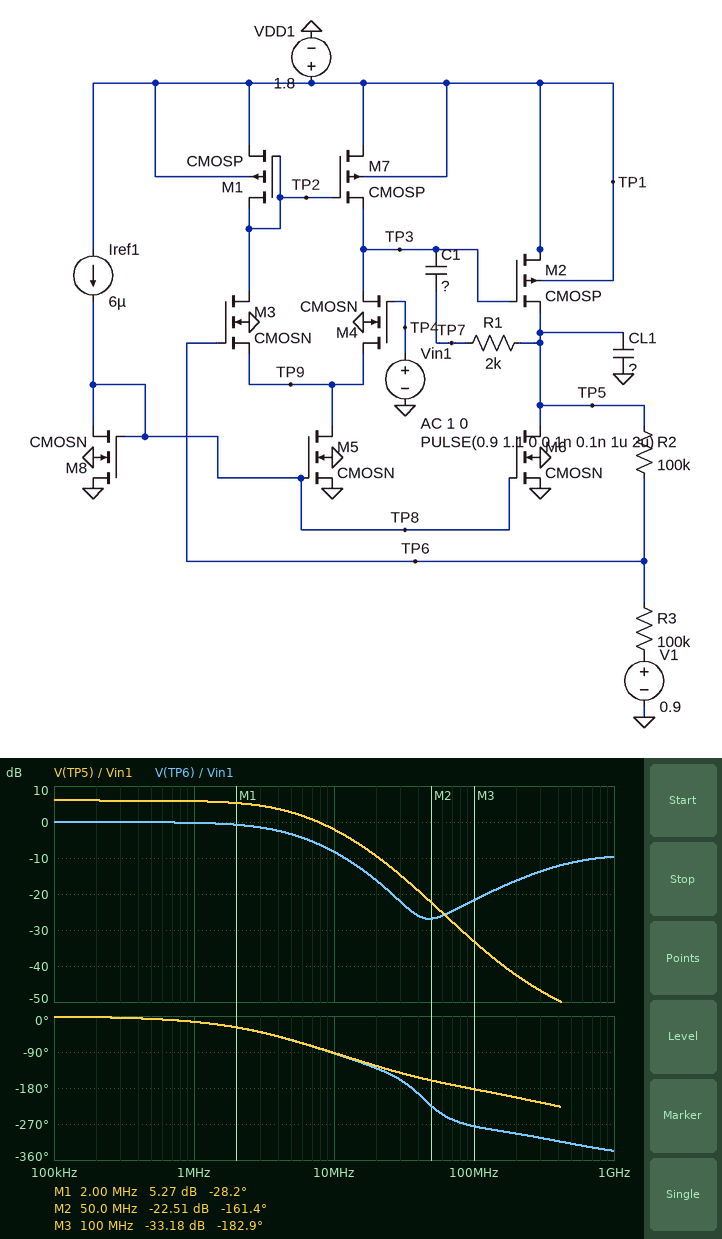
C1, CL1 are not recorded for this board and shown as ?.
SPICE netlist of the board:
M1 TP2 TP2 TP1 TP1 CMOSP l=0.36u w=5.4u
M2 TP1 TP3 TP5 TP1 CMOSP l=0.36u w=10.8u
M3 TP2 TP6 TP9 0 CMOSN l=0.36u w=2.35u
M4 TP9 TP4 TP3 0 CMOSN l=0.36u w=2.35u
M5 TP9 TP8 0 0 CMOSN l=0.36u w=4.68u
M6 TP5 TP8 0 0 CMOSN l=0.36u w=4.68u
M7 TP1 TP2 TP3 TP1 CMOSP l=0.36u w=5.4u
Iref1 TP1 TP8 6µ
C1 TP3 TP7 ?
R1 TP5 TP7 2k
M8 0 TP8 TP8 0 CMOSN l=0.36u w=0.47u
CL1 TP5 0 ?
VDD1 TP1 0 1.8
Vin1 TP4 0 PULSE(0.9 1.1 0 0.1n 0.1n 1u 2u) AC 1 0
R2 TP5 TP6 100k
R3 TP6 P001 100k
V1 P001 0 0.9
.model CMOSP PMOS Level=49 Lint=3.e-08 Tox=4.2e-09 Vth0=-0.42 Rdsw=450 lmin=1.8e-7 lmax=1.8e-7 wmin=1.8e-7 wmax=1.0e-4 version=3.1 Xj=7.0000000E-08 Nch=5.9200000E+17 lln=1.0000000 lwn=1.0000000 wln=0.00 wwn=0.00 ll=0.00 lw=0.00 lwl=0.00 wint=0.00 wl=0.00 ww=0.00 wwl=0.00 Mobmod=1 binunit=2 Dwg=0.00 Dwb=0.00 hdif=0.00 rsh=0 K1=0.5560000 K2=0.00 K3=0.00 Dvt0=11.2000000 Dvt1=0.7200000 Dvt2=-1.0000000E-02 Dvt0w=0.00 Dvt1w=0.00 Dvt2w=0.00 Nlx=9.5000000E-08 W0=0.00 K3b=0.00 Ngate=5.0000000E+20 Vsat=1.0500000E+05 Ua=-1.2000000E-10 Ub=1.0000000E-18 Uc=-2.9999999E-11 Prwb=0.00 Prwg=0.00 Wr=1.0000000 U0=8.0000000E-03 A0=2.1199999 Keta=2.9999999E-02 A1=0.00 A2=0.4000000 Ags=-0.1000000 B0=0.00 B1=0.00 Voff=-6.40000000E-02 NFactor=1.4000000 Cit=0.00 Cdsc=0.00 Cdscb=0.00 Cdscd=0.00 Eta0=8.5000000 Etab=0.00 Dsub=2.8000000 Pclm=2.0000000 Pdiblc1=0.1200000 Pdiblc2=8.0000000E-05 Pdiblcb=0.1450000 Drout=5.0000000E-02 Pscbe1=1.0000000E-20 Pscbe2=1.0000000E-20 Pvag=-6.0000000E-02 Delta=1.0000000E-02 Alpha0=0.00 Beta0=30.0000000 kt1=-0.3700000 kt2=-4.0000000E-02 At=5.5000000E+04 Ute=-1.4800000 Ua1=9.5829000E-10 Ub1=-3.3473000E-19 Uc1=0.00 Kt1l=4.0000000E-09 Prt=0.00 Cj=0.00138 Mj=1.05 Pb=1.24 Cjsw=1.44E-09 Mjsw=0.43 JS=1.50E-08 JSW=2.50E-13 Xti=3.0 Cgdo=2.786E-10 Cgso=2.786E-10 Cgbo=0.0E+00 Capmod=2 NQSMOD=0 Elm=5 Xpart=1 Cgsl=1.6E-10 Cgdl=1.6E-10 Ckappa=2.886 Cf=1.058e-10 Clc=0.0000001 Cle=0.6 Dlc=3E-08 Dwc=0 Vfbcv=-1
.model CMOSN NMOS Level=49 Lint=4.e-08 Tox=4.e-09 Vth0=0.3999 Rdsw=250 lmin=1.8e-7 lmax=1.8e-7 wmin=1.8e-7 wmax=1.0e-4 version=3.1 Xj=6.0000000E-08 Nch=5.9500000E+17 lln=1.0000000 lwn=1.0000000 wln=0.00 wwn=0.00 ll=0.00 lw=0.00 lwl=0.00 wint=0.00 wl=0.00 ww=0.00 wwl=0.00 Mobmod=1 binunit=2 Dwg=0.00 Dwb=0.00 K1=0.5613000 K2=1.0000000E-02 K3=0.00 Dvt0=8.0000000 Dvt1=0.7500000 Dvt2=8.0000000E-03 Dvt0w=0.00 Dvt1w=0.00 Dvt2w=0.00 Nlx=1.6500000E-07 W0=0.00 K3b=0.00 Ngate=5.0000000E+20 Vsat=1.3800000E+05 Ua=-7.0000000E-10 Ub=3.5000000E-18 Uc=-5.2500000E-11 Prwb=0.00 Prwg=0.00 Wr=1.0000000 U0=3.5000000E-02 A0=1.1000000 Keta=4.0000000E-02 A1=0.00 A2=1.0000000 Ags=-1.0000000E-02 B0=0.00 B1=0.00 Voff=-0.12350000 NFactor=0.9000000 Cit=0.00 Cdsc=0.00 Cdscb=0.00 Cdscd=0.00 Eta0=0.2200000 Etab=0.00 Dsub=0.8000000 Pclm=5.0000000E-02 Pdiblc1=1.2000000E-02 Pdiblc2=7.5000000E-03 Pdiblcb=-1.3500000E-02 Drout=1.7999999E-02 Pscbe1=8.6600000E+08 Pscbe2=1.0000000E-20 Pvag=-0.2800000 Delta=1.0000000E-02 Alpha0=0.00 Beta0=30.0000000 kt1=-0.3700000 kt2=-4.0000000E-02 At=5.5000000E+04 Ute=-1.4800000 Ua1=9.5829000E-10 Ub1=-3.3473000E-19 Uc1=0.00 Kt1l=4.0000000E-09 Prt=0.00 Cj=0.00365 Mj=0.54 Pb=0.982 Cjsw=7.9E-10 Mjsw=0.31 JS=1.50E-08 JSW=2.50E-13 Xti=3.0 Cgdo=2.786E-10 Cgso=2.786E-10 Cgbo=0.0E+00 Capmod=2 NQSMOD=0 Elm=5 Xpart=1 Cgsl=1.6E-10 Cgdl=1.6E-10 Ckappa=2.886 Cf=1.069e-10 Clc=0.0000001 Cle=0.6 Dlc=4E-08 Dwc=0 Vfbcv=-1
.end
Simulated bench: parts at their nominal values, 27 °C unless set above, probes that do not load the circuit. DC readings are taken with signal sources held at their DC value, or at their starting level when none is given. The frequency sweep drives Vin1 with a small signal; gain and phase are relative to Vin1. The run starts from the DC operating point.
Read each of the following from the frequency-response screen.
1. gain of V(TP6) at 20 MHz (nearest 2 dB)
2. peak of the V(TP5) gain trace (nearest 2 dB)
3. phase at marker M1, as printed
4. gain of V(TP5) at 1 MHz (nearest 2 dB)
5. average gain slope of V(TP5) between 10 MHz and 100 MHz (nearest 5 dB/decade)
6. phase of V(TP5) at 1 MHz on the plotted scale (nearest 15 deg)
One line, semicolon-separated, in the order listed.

-16 dB; 6 dB; -28.2 deg; 6 dB; -30 dB/decade; -15 deg
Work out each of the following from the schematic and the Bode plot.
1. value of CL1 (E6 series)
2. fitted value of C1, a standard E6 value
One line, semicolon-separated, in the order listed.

3.3 pF; 4.7 pF
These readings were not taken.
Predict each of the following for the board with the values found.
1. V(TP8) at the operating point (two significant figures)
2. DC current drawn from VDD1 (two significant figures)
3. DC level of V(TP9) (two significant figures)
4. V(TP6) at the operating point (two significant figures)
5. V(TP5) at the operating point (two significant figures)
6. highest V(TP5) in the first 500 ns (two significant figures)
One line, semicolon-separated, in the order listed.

680 mV; 120 µA; 180 mV; 900 mV; 900 mV; 1.3 V
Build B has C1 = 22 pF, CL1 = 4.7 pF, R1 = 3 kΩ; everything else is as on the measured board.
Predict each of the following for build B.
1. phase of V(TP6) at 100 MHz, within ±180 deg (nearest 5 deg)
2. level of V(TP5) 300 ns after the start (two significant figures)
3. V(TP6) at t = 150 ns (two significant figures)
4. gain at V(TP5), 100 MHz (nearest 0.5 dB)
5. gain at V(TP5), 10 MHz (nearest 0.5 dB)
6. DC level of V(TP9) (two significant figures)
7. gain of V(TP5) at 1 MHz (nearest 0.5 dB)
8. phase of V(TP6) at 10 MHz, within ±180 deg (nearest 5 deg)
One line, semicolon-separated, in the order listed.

80 deg; 1.2 V; 1.0 V; -28.5 dB; -12.5 dB; 180 mV; 2.0 dB; -60 deg
